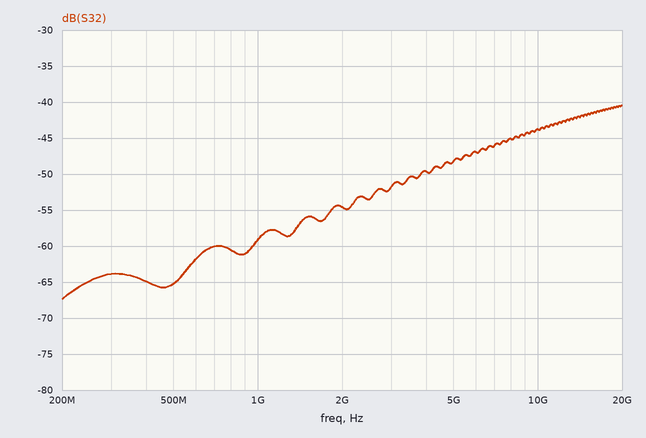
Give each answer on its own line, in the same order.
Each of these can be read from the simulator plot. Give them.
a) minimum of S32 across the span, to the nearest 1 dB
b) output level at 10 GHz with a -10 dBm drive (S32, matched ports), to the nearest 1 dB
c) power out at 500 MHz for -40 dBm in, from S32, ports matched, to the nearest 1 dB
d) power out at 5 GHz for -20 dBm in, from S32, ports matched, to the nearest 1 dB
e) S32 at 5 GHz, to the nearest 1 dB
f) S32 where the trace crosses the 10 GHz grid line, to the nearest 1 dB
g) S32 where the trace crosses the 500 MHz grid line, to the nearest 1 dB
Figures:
-67 dB
-54 dBm
-105 dBm
-68 dBm
-48 dB
-44 dB
-65 dB
